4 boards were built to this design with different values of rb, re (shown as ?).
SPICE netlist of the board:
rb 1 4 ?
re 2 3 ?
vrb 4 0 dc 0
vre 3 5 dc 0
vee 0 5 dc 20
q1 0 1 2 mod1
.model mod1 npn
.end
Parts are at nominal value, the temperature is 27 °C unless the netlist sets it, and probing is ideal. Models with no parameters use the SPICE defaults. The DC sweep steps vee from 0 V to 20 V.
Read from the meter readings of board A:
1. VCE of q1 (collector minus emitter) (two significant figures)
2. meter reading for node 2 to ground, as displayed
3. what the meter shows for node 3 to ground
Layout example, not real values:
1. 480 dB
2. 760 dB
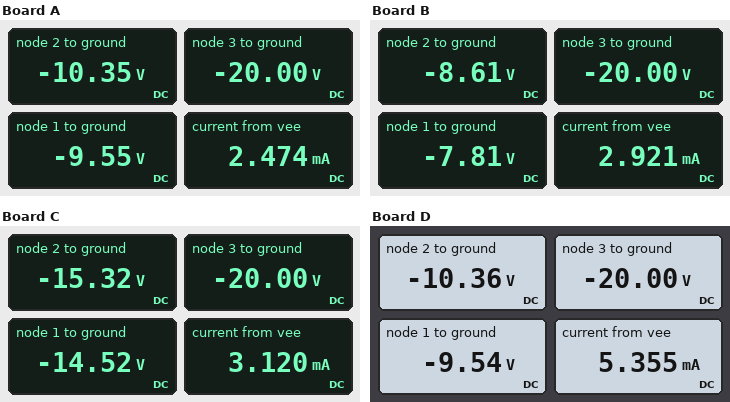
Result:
1. 10 V
2. -10.35 V
3. -20.00 V
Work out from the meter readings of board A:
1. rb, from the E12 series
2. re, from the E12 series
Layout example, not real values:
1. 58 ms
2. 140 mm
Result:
1. 390 kΩ
2. 3.9 kΩ
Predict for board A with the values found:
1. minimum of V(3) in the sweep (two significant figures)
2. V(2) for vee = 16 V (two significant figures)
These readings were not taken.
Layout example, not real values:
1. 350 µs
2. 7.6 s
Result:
1. -20 V
2. -8.4 V
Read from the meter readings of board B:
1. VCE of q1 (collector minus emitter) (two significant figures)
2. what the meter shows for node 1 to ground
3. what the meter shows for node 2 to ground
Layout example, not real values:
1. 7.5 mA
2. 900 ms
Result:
1. 8.6 V
2. -7.81 V
3. -8.61 V
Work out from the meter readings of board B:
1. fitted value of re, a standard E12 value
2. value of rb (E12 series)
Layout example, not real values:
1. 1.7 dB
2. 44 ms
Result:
1. 3.9 kΩ
2. 270 kΩ
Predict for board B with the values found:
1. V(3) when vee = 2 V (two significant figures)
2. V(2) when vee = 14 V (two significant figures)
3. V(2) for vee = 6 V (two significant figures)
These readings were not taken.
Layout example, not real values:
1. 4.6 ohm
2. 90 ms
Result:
1. -2.0 V
2. -6.2 V
3. -2.9 V
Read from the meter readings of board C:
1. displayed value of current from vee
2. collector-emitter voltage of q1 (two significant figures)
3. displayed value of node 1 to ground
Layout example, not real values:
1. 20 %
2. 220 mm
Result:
1. 3.120 mA
2. 15 V
3. -14.52 V
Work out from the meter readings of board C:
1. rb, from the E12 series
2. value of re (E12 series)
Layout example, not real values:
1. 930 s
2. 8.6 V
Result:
1. 470 kΩ
2. 1.5 kΩ
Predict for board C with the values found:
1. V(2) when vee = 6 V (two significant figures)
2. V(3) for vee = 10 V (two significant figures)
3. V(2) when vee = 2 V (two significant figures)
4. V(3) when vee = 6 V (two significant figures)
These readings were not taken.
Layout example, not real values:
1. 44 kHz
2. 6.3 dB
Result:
1. -4.7 V
2. -10 V
3. -1.7 V
4. -6.0 V
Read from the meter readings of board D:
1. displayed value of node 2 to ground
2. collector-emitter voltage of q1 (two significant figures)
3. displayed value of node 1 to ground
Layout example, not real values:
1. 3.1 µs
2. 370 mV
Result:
1. -10.36 V
2. 10 V
3. -9.54 V
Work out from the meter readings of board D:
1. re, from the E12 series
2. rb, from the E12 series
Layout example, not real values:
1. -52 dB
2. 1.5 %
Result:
1. 1.8 kΩ
2. 180 kΩ
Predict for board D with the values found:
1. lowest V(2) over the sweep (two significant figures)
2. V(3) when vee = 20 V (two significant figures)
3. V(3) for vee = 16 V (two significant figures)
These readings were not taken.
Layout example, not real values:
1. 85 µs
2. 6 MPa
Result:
1. -10 V
2. -20 V
3. -16 V
